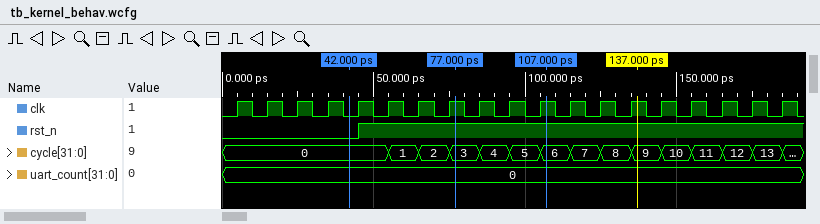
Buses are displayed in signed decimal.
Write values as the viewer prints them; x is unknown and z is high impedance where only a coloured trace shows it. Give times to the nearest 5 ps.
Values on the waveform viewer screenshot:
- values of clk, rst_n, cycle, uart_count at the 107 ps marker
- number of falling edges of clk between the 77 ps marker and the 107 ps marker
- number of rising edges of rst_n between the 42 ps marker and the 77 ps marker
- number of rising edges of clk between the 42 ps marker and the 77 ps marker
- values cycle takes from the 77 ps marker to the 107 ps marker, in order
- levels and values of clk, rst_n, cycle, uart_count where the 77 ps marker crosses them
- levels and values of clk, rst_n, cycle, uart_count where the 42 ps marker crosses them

clk=1, rst_n=1, cycle=6, uart_count=0
3
1
4
3, 4, 5, 6
clk=1, rst_n=1, cycle=3, uart_count=0
clk=0, rst_n=0, cycle=0, uart_count=0
